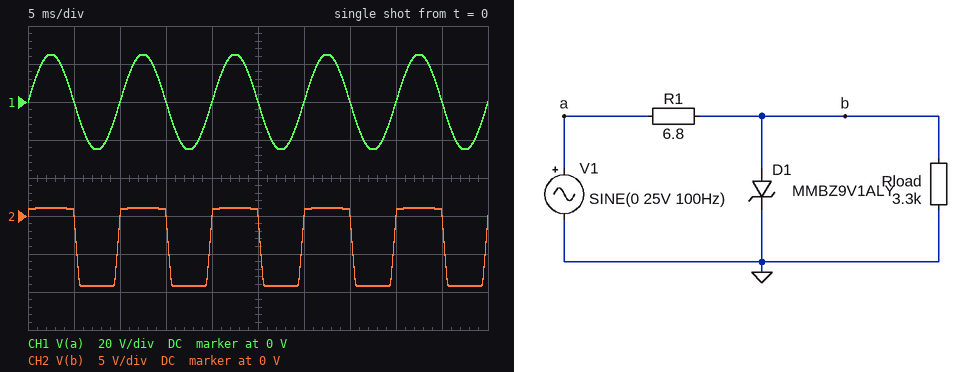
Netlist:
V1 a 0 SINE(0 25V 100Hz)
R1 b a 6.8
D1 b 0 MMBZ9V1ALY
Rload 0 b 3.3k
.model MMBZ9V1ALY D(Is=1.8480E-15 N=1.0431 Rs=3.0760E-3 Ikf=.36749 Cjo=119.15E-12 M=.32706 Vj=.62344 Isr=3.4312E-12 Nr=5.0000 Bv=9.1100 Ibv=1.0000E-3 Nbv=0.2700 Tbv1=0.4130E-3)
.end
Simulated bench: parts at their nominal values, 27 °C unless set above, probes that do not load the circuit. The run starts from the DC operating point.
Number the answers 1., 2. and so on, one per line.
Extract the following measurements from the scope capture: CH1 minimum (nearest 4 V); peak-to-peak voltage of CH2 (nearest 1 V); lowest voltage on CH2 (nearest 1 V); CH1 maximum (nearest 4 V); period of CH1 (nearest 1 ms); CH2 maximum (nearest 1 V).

1. -24 V
2. 10 V
3. -9 V
4. 24 V
5. 10 ms
6. 1 V
